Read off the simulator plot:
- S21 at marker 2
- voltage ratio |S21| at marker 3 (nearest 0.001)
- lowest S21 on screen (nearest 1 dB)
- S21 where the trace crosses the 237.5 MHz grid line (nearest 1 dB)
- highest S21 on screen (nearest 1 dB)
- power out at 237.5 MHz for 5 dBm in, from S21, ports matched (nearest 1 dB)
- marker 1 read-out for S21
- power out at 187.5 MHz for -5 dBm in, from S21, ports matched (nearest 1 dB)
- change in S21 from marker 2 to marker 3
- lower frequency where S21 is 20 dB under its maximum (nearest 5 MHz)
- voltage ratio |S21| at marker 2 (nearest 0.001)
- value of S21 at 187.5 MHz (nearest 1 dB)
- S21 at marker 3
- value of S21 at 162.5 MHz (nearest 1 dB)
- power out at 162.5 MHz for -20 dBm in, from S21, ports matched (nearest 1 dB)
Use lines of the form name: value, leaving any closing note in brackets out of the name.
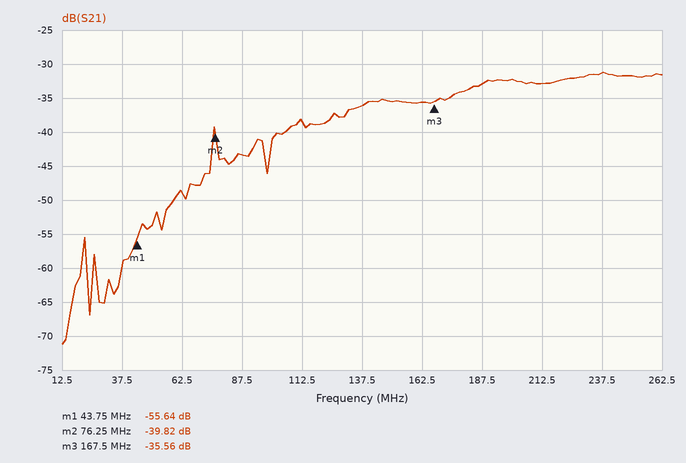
S21 at marker 2: -39.82 dB
voltage ratio |S21| at marker 3: 0.017
lowest S21 on screen: -71 dB
S21 where the trace crosses the 237.5 MHz grid line: -31 dB
highest S21 on screen: -31 dB
power out at 237.5 MHz for 5 dBm in, from S21, ports matched: -26 dBm
marker 1 read-out for S21: -55.64 dB
power out at 187.5 MHz for -5 dBm in, from S21, ports matched: -38 dBm
change in S21 from marker 2 to marker 3: 4.26 dB
lower frequency where S21 is 20 dB under its maximum: 55 MHz
voltage ratio |S21| at marker 2: 0.010
value of S21 at 187.5 MHz: -33 dB
S21 at marker 3: -35.56 dB
value of S21 at 162.5 MHz: -36 dB
power out at 162.5 MHz for -20 dBm in, from S21, ports matched: -56 dBm
